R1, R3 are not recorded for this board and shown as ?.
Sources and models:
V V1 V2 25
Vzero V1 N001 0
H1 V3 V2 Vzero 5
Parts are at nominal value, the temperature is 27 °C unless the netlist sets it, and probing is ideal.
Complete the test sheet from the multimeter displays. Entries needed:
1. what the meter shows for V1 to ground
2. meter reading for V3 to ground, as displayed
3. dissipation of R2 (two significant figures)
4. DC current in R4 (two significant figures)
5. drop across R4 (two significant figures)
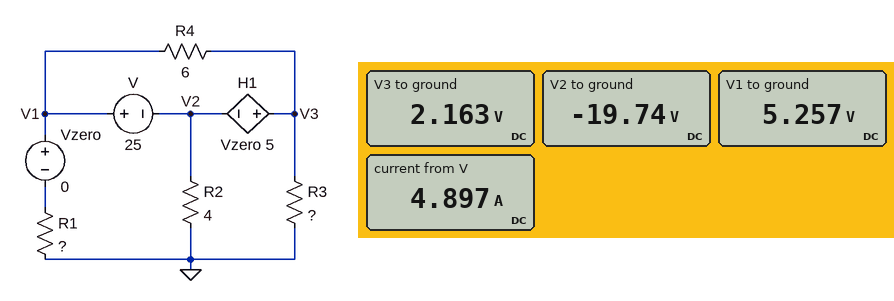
5.257 V
2.163 V
97 W
520 mA
3.1 V
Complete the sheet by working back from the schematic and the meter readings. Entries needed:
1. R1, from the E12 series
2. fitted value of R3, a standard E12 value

1.2 Ω
3.9 Ω
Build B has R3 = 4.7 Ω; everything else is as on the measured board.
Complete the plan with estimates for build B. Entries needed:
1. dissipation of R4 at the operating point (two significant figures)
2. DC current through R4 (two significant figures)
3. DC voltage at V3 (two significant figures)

1.4 W
490 mA
2.4 V
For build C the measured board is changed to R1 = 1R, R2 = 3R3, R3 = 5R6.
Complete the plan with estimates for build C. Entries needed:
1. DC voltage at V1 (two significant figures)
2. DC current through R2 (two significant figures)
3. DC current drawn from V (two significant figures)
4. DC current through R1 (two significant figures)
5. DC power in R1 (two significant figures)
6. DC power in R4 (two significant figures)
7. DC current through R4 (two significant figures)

5.1 V
6.0 A
5.0 A
5.1 A
26 W
21 mW
59 mA
